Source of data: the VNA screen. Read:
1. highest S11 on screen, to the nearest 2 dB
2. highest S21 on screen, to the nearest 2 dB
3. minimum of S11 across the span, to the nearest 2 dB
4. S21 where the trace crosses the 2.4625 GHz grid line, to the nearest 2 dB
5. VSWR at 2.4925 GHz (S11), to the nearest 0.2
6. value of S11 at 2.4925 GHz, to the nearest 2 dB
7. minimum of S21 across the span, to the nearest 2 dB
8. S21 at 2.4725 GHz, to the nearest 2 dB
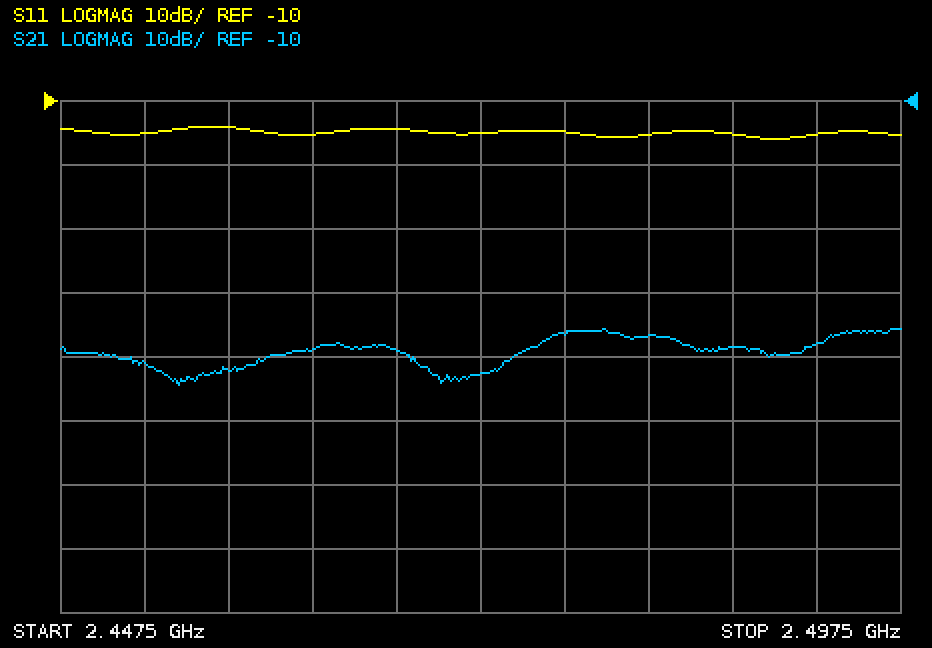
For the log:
-14 dB
-46 dB
-16 dB
-48 dB
1.4
-16 dB
-54 dB
-52 dB
